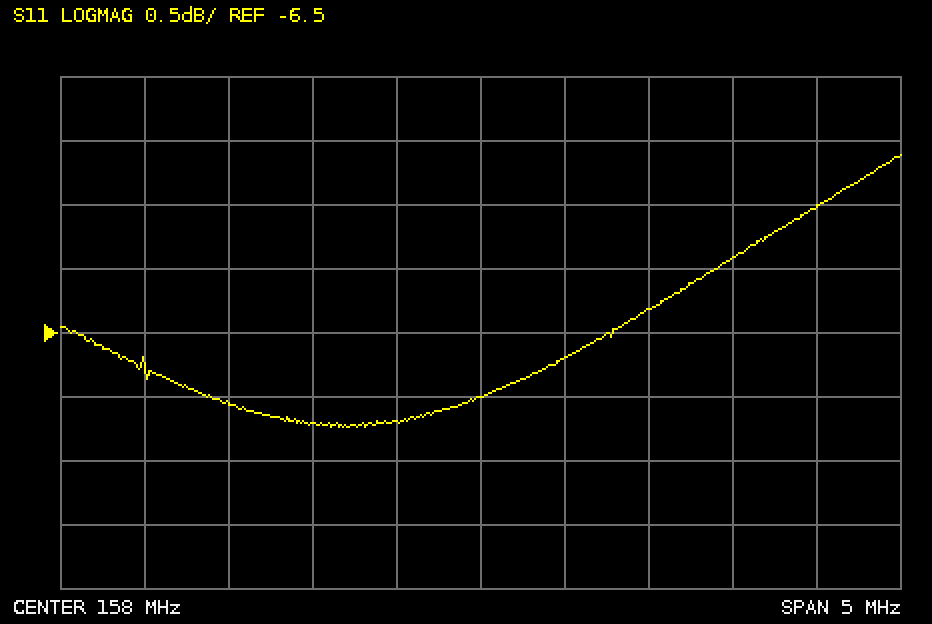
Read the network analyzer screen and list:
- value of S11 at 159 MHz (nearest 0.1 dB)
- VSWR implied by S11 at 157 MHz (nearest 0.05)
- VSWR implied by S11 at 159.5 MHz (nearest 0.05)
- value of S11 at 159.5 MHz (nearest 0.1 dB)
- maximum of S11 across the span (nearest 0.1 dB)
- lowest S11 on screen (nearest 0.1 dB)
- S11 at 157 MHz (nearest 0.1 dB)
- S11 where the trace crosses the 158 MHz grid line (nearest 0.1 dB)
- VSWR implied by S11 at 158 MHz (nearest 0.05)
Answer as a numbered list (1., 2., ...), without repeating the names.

1. -6.3 dB
2. 2.55
3. 3.05
4. -5.9 dB
5. -5.1 dB
6. -7.2 dB
7. -7.2 dB
8. -7.0 dB
9. 2.60
